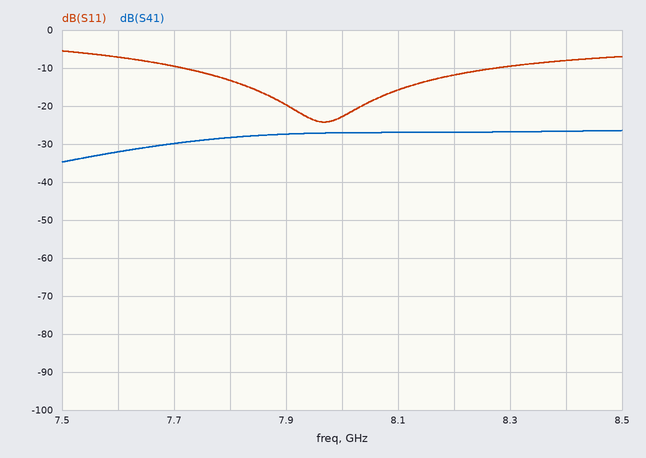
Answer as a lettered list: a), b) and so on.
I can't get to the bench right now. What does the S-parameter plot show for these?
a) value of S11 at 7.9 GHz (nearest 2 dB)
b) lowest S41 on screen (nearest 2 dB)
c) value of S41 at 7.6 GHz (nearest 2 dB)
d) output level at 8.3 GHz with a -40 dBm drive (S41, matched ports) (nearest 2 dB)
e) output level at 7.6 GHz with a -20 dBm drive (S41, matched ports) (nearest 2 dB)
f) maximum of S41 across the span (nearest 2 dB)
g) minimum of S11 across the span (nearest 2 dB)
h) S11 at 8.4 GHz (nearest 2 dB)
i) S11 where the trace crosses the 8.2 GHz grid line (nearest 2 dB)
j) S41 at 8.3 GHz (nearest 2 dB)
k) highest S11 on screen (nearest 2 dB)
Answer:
a) -20 dB
b) -34 dB
c) -32 dB
d) -66 dBm
e) -52 dBm
f) -26 dB
g) -24 dB
h) -8 dB
i) -12 dB
j) -26 dB
k) -6 dB
